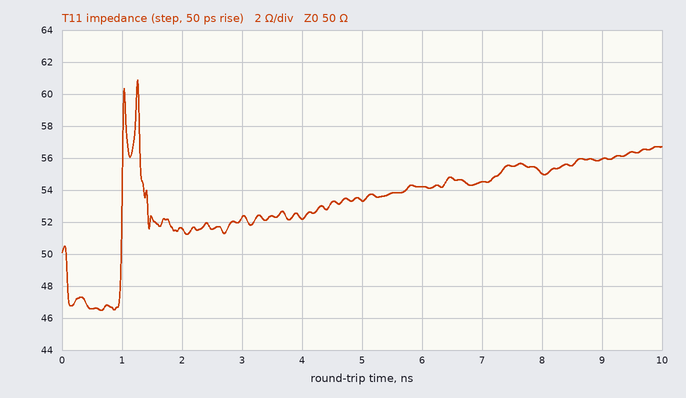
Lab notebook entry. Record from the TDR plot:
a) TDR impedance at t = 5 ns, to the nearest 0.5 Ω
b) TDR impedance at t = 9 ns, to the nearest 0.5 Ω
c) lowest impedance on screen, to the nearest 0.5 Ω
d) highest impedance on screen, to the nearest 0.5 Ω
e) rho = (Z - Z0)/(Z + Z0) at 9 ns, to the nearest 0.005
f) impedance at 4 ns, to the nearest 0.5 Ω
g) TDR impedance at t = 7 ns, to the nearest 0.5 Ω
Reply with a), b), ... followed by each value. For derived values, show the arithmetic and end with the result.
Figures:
a) 53.5 Ω
b) 56.0 Ω
c) 46.5 Ω
d) 61.0 Ω
e) (56 − 50)/(56 + 50) ≈ +0.0566, so +0.055 to the nearest 0.005
f) 52.0 Ω
g) 54.5 Ω
